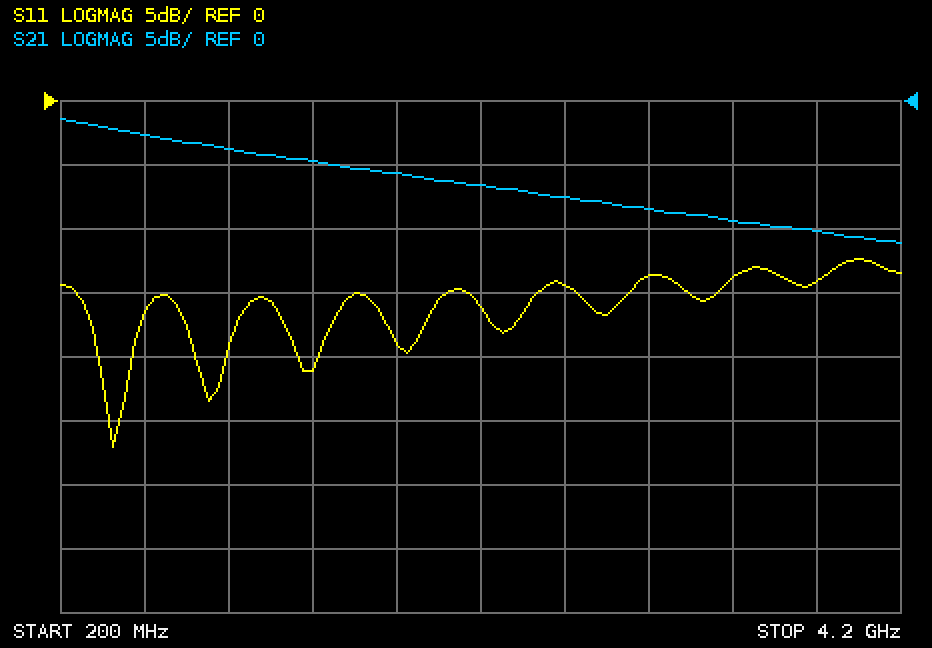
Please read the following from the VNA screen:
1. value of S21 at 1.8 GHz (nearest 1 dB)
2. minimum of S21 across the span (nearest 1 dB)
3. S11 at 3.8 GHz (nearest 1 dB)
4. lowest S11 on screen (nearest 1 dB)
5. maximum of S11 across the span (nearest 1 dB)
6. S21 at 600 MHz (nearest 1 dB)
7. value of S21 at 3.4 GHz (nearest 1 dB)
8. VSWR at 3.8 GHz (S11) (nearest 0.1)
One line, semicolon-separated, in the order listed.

-6 dB; -11 dB; -14 dB; -27 dB; -12 dB; -3 dB; -9 dB; 1.5
